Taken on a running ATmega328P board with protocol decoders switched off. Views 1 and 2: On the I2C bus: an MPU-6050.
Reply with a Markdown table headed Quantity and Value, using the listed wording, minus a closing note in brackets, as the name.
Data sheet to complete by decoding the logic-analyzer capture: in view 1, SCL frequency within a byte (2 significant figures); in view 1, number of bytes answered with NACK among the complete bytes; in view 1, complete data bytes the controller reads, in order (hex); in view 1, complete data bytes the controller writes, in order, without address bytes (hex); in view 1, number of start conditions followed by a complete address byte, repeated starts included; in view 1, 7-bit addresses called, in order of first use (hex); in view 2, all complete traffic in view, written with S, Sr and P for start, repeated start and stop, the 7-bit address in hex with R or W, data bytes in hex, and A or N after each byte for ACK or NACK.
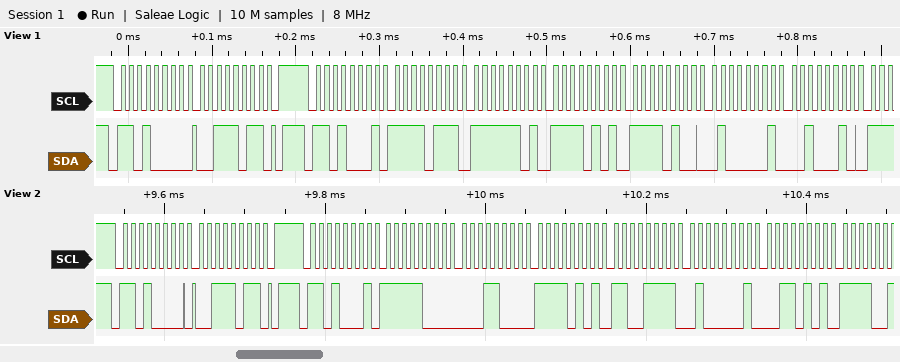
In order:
| Quantity | Value |
|---|---|
| in view 1, SCL frequency within a byte | 100 kHz |
| in view 1, number of bytes answered with NACK among the complete bytes | 0 |
| in view 1, complete data bytes the controller reads, in order | F7 FD F5 F4 41 22 |
| in view 1, complete data bytes the controller writes, in order, without address bytes | 3B |
| in view 1, number of start conditions followed by a complete address byte, repeated starts included | 2 |
| in view 1, 7-bit addresses called, in order of first use | 0x68 |
| in view 2, all complete traffic in view, written with S, Sr and P for start, repeated start and stop, the 7-bit address in hex with R or W, data bytes in hex, and A or N after each byte for ACK or NACK | S 68W A 3B A P S 68R A F8 A 18 A F5 A CF A 41 A 35 A |
